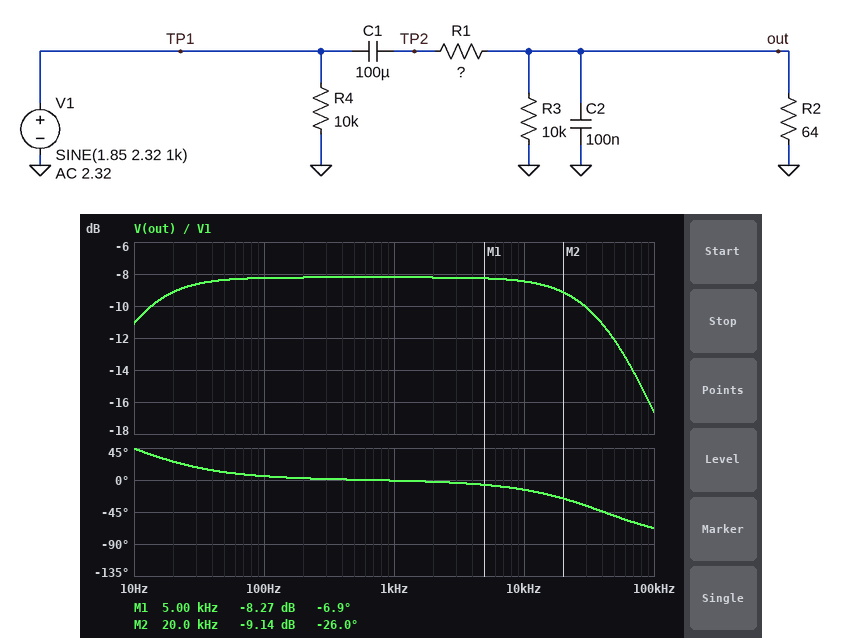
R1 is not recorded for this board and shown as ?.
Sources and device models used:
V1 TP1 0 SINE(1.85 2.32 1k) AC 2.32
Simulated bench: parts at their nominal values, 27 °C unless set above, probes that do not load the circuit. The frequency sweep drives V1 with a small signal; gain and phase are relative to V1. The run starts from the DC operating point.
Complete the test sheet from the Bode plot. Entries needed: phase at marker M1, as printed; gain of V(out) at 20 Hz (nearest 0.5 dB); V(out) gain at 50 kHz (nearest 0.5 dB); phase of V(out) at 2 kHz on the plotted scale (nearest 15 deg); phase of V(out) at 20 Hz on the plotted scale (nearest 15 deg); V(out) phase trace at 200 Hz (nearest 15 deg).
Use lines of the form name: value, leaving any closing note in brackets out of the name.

phase at marker M1, as printed: -6.9 deg
gain of V(out) at 20 Hz: -9.0 dB
V(out) gain at 50 kHz: -12.0 dB
phase of V(out) at 2 kHz on the plotted scale: 0 deg
phase of V(out) at 20 Hz on the plotted scale: 30 deg
V(out) phase trace at 200 Hz: 0 deg
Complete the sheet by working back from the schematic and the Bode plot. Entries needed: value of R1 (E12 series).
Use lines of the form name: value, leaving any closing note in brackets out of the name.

value of R1: 100 Ω
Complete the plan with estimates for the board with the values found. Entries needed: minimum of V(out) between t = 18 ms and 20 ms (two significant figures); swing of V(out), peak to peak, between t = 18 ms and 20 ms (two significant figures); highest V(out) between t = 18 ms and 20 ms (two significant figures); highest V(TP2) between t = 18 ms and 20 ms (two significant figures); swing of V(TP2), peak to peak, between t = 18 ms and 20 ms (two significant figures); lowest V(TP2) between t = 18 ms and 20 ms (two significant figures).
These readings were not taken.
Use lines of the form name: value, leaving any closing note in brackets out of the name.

minimum of V(out) between t = 18 ms and 20 ms: -900 mV
swing of V(out), peak to peak, between t = 18 ms and 20 ms: 1.8 V
highest V(out) between t = 18 ms and 20 ms: 900 mV
highest V(TP2) between t = 18 ms and 20 ms: 2.3 V
swing of V(TP2), peak to peak, between t = 18 ms and 20 ms: 4.6 V
lowest V(TP2) between t = 18 ms and 20 ms: -2.3 V
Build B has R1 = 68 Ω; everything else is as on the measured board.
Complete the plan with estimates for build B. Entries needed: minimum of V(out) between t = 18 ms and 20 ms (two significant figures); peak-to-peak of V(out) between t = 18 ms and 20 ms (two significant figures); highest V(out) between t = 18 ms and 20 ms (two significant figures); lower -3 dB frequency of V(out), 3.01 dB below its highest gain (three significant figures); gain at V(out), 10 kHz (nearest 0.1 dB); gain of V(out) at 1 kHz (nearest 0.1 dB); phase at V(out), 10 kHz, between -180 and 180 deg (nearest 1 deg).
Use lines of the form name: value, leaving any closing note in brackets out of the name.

minimum of V(out) between t = 18 ms and 20 ms: -1.1 V
peak-to-peak of V(out) between t = 18 ms and 20 ms: 2.2 V
highest V(out) between t = 18 ms and 20 ms: 1.1 V
lower -3 dB frequency of V(out), 3.01 dB below its highest gain: 12.1 Hz
gain at V(out), 10 kHz: -6.5 dB
gain of V(out) at 1 kHz: -6.3 dB
phase at V(out), 10 kHz, between -180 and 180 deg: -12 deg
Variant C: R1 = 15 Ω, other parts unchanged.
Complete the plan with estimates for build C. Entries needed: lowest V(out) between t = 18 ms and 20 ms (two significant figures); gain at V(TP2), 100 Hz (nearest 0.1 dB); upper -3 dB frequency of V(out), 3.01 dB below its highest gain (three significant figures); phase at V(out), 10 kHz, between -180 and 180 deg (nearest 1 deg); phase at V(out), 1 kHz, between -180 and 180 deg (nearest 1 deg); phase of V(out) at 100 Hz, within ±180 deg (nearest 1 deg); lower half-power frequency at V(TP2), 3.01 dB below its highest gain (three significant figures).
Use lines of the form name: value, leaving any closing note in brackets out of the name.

lowest V(out) between t = 18 ms and 20 ms: -1.9 V
gain at V(TP2), 100 Hz: -0.2 dB
upper -3 dB frequency of V(out), 3.01 dB below its highest gain: 131 kHz
phase at V(out), 10 kHz, between -180 and 180 deg: -4 deg
phase at V(out), 1 kHz, between -180 and 180 deg: 1 deg
phase of V(out) at 100 Hz, within ±180 deg: 11 deg
lower half-power frequency at V(TP2), 3.01 dB below its highest gain: 20.3 Hz
